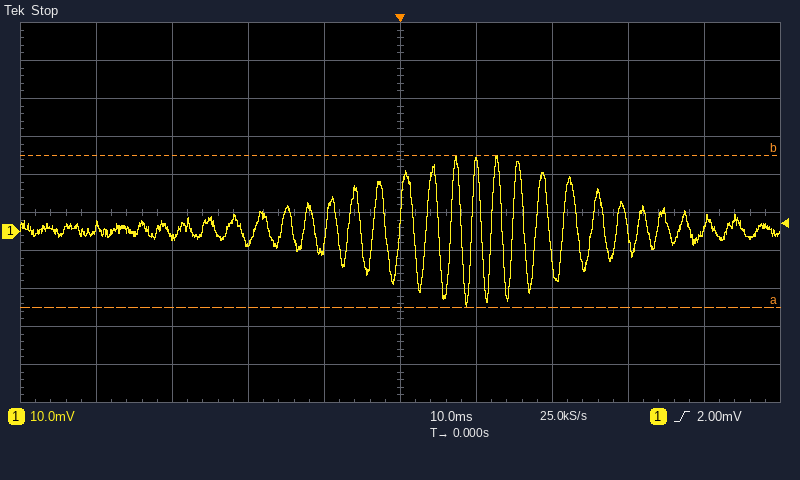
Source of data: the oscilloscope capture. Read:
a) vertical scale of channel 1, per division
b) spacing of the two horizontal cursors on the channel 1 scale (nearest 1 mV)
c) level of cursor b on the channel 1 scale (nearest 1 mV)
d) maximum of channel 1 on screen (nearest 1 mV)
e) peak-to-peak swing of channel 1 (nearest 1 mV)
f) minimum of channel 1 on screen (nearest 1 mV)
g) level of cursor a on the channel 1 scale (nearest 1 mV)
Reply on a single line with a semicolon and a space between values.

10 mV; 40 mV; 20 mV; 20 mV; 40 mV; -20 mV; -20 mV
